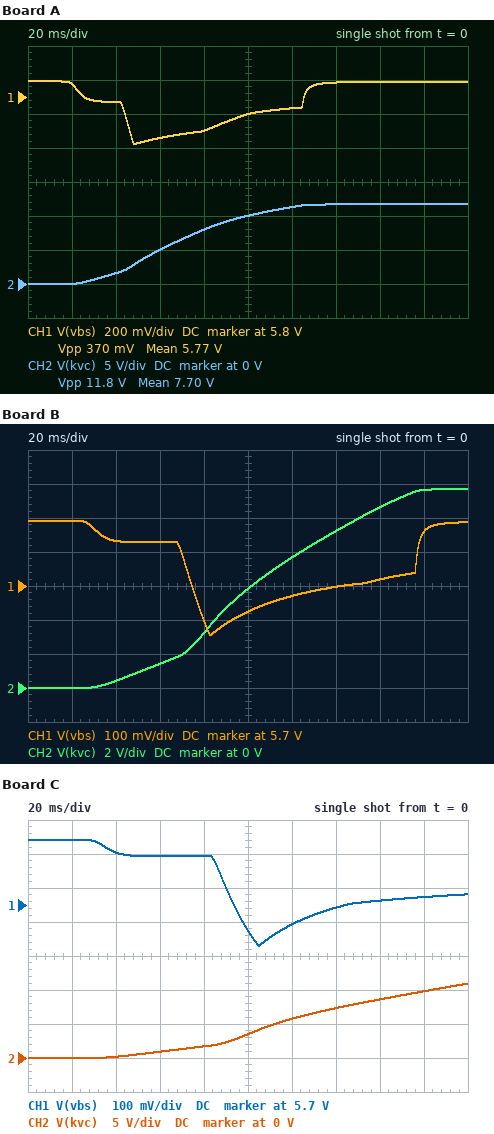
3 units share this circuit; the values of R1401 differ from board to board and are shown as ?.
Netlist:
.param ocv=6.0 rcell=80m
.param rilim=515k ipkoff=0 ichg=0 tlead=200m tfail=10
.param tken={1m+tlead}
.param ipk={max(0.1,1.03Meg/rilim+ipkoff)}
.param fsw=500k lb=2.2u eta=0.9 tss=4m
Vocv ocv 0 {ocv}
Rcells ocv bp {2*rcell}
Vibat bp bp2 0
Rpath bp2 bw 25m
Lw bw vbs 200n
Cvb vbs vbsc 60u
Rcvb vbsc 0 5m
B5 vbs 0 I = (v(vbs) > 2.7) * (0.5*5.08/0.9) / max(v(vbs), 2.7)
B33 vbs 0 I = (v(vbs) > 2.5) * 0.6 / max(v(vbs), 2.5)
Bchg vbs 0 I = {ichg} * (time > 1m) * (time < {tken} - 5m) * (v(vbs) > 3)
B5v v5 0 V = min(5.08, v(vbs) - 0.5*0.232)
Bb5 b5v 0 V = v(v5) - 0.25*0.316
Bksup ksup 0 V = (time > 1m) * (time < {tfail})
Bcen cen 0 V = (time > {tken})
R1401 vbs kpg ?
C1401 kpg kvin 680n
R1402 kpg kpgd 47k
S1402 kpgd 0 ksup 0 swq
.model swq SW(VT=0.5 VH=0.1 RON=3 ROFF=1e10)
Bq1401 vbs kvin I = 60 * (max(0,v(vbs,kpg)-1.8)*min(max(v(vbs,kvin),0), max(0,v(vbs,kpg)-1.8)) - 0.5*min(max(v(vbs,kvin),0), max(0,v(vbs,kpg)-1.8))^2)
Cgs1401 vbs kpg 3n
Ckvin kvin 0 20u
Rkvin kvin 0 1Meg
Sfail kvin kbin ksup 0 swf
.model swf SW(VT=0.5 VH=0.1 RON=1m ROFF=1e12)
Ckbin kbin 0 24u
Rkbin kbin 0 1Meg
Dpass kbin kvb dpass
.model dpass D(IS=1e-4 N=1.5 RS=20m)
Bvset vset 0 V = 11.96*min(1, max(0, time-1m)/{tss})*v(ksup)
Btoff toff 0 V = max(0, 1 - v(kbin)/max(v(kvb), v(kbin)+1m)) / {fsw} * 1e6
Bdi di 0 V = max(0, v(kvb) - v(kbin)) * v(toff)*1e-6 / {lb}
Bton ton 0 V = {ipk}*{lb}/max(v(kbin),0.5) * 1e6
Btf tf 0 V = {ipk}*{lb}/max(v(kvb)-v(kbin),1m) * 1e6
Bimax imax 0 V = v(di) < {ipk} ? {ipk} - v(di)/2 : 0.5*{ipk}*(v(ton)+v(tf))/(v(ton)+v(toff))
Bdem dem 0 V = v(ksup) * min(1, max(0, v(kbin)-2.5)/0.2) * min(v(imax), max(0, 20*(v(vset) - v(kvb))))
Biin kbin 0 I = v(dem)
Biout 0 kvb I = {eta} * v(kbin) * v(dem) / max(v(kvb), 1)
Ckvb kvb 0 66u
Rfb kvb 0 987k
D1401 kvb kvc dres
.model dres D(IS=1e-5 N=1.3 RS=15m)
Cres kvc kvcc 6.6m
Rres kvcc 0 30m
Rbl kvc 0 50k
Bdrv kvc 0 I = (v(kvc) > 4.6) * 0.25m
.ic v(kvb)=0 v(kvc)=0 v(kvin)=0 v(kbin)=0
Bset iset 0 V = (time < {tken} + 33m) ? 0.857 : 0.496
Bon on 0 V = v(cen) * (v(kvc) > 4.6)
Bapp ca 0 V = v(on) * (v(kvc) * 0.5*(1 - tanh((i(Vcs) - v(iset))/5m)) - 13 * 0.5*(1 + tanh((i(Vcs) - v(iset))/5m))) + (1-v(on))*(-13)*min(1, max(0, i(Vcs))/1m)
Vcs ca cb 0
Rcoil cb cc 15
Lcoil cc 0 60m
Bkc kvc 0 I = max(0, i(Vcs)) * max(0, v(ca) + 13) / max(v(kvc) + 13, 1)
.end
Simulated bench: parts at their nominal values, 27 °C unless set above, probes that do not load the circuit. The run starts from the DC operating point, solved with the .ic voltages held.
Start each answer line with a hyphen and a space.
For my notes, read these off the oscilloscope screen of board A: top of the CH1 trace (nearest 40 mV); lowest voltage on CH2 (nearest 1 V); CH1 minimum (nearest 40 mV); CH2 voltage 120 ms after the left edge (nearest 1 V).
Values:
- 5.88 V
- 0 V
- 5.52 V
- 11 V
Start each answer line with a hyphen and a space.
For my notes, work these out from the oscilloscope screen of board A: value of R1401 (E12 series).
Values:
- 120 kΩ
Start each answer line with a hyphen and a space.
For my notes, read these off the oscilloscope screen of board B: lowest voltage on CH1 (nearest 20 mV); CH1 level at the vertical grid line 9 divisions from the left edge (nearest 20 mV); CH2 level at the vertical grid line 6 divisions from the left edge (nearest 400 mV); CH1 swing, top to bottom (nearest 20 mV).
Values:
- 5.56 V
- 5.86 V
- 7.6 V
- 340 mV
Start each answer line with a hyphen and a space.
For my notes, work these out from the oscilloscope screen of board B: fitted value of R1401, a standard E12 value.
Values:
- 39 kΩ
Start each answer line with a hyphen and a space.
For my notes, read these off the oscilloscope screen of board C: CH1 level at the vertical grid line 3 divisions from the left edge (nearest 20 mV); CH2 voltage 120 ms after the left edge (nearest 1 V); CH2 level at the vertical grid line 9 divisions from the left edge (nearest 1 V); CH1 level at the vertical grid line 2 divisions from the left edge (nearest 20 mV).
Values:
- 5.84 V
- 6 V
- 10 V
- 5.86 V
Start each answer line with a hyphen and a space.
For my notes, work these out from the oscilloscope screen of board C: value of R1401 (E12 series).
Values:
- 33 kΩ
